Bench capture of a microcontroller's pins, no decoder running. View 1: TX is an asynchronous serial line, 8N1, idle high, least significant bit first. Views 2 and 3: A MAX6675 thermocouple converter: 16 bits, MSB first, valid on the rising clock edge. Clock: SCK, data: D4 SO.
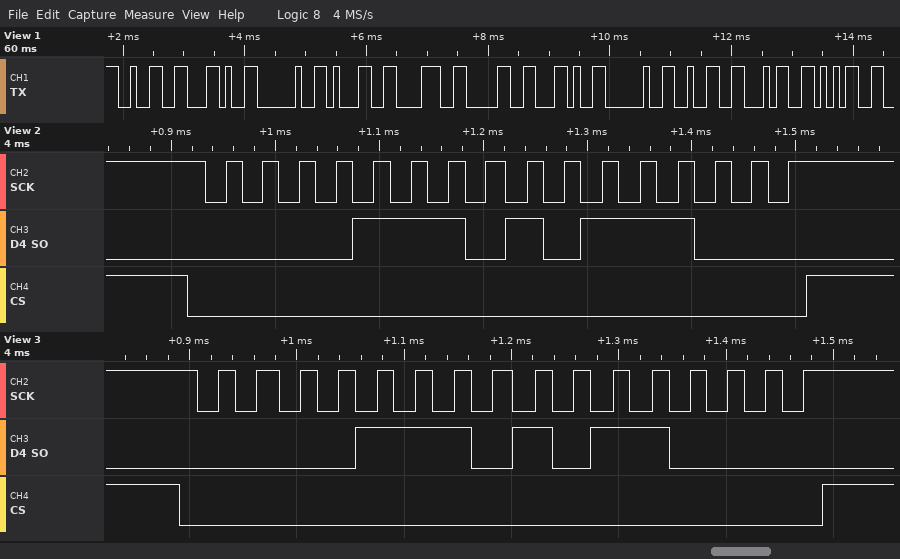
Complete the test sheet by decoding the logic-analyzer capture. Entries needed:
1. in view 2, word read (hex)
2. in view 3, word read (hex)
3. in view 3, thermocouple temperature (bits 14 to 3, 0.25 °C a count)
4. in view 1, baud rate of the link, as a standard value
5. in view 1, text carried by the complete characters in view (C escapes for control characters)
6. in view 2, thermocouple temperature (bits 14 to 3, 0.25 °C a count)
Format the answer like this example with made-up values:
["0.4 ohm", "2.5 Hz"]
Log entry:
["0x0EB8", "0x0EB0", "117.50 °C", "9600 baud", "\"2, 180, 245\"", "117.75 °C"]
